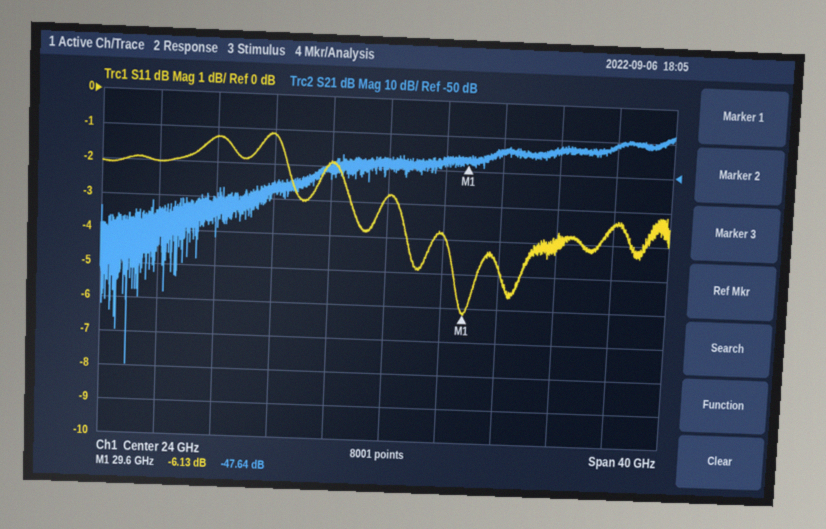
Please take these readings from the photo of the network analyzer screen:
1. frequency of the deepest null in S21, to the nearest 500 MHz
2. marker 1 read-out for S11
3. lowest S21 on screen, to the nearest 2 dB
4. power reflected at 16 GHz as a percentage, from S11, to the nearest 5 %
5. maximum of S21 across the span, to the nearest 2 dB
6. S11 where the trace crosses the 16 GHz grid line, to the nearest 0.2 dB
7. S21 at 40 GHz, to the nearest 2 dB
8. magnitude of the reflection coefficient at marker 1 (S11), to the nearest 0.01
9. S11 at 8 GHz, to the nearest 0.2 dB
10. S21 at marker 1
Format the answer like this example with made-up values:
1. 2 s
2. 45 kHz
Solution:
1. 6.0 GHz
2. -6.13 dB
3. -110 dB
4. 75 %
5. -38 dB
6. -1.2 dB
7. -42 dB
8. 0.49
9. -2.0 dB
10. -47.64 dB
